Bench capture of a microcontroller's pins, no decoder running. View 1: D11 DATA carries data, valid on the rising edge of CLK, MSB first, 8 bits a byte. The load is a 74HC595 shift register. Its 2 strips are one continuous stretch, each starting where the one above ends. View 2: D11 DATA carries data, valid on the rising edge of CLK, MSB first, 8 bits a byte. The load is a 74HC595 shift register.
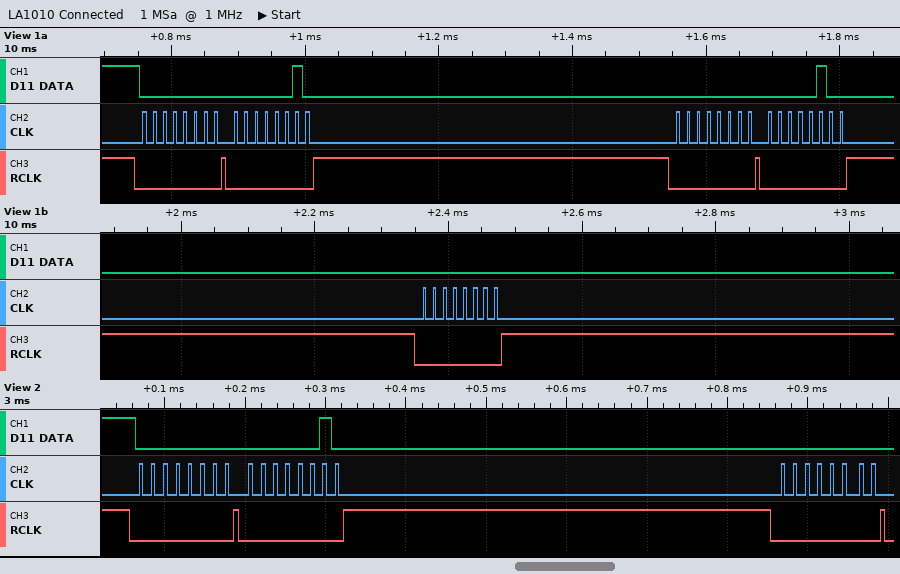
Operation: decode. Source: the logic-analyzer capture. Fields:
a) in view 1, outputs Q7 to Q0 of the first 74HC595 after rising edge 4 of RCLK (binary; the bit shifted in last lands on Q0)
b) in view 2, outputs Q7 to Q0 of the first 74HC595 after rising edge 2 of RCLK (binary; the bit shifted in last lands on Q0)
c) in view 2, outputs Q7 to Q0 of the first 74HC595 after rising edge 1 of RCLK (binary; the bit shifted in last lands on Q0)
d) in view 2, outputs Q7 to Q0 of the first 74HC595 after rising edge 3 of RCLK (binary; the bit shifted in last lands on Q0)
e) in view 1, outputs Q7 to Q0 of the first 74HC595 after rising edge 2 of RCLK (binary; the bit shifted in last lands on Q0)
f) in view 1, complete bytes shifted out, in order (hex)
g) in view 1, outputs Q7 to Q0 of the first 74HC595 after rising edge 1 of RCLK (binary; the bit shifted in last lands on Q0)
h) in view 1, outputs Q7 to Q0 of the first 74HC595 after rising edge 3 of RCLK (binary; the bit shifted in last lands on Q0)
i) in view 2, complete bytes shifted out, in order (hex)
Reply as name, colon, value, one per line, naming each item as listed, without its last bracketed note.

in view 1, outputs Q7 to Q0 of the first 74HC595 after rising edge 4 of RCLK: 00000100
in view 2, outputs Q7 to Q0 of the first 74HC595 after rising edge 2 of RCLK: 00000010
in view 2, outputs Q7 to Q0 of the first 74HC595 after rising edge 1 of RCLK: 00000000
in view 2, outputs Q7 to Q0 of the first 74HC595 after rising edge 3 of RCLK: 00000000
in view 1, outputs Q7 to Q0 of the first 74HC595 after rising edge 2 of RCLK: 00000010
in view 1, complete bytes shifted out, in order: 0x00 0x02 0x00 0x04 0x00
in view 1, outputs Q7 to Q0 of the first 74HC595 after rising edge 1 of RCLK: 00000000
in view 1, outputs Q7 to Q0 of the first 74HC595 after rising edge 3 of RCLK: 00000000
in view 2, complete bytes shifted out, in order: 00 02 00
